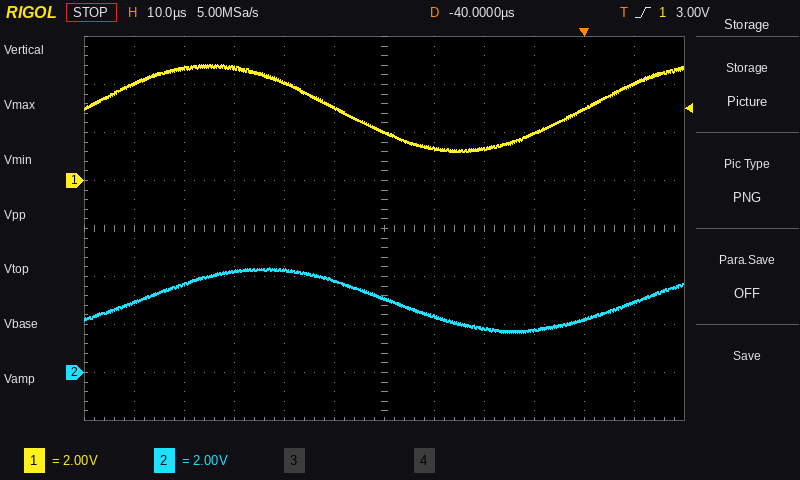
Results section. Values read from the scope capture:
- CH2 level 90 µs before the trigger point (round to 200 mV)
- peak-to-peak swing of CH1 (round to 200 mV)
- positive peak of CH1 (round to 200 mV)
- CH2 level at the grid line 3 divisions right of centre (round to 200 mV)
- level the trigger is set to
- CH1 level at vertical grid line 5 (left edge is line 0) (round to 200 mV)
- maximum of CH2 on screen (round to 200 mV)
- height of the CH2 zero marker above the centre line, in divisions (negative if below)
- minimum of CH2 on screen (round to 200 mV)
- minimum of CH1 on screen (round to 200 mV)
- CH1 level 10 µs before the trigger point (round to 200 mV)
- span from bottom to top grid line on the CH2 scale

3.0 V
3.6 V
4.8 V
1.8 V
3.00 V
3.0 V
4.4 V
-3.0 div
1.6 V
1.2 V
2.0 V
16 V
